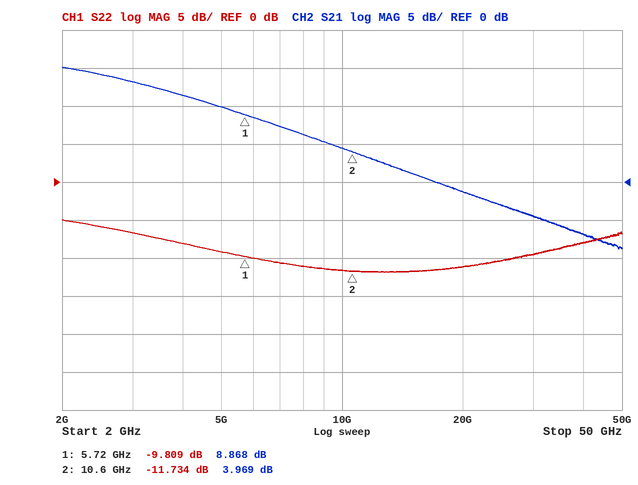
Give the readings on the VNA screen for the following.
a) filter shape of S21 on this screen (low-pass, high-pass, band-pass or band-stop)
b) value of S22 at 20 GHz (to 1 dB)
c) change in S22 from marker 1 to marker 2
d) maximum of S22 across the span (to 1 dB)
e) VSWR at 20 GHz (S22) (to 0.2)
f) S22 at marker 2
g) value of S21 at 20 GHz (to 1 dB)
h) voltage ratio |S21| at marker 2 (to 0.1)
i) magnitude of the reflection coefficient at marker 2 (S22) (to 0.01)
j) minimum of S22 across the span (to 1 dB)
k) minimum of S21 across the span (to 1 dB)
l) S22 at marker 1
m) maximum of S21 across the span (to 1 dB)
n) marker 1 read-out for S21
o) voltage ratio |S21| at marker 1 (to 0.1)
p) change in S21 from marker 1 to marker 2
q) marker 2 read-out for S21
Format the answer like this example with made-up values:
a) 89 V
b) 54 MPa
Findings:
a) low-pass
b) -11 dB
c) -1.925 dB
d) -5 dB
e) 1.8
f) -11.734 dB
g) -1 dB
h) 1.6
i) 0.26
j) -12 dB
k) -9 dB
l) -9.809 dB
m) 15 dB
n) 8.868 dB
o) 2.8
p) -4.899 dB
q) 3.969 dB
